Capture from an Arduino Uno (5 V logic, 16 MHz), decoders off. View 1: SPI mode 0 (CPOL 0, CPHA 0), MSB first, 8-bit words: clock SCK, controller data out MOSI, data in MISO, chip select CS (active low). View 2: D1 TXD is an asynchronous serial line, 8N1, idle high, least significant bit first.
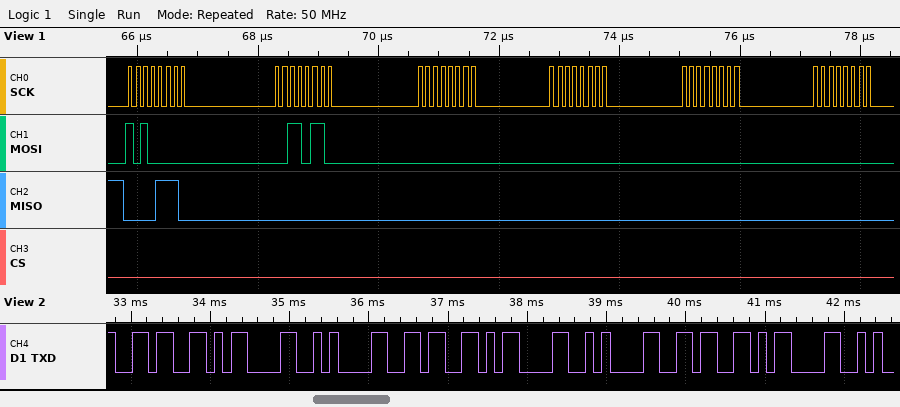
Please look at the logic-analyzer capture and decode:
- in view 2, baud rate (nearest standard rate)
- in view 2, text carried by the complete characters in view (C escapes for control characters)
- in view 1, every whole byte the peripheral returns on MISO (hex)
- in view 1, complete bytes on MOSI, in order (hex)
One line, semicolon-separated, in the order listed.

9600 baud; "6\r\n6\r\n6\r"; 0x0E 0x00 0x00 0x00 0x00 0x00; 0xA0 0x36 0x00 0x00 0x00 0x00
